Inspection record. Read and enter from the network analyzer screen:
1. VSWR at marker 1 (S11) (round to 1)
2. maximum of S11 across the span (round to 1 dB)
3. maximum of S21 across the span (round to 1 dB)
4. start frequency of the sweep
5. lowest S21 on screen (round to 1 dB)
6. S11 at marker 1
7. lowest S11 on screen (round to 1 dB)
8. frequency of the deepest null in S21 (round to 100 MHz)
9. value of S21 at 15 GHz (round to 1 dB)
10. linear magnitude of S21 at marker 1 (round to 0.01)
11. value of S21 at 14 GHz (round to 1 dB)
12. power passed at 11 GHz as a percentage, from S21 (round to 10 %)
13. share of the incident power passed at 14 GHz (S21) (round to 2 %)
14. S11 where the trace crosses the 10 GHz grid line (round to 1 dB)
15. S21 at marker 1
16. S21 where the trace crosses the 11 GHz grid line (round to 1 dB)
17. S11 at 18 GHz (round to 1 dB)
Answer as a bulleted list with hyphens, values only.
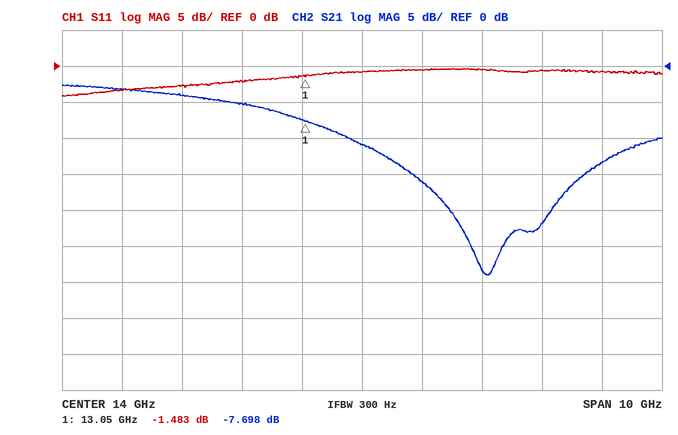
- 12
- 0 dB
- -3 dB
- 9 GHz
- -29 dB
- -1.483 dB
- -4 dB
- 16.1 GHz
- -16 dB
- 0.41
- -11 dB
- 40 %
- 8 %
- -3 dB
- -7.698 dB
- -4 dB
- -1 dB
